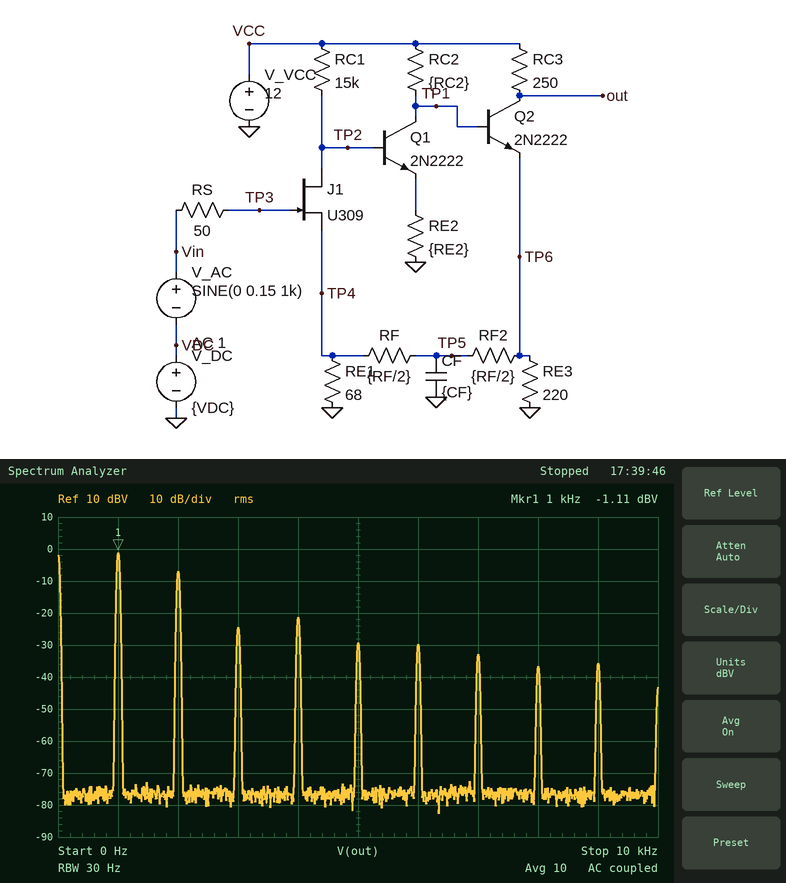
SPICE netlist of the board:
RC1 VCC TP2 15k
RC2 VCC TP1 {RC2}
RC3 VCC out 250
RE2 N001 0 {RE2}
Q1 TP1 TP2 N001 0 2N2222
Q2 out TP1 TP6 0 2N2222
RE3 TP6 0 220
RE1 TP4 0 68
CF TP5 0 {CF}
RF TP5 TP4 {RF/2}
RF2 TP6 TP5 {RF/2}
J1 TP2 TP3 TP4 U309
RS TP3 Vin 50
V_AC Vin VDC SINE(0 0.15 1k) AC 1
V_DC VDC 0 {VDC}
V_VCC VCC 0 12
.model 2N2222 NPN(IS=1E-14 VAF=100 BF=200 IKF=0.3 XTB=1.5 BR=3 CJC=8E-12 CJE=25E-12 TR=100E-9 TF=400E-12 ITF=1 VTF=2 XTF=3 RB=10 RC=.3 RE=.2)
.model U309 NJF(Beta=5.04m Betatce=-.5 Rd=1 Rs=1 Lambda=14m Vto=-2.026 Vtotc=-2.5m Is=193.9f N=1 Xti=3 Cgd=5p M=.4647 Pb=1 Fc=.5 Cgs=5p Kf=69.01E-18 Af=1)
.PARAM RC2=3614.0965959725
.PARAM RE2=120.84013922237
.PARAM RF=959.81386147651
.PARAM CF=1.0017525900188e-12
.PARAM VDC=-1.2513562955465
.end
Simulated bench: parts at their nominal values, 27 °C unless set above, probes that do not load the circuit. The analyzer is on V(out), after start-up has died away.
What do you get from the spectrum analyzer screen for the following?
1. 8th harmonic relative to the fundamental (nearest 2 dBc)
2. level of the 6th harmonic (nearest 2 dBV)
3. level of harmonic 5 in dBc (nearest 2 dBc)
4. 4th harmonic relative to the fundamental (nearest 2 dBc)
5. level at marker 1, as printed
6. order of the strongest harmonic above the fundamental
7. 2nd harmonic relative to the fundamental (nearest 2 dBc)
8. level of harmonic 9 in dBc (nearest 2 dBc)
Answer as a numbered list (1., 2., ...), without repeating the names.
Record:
1. -36 dBc
2. -30 dBV
3. -28 dBc
4. -20 dBc
5. -1.11 dBV
6. 2
7. -6 dBc
8. -34 dBc
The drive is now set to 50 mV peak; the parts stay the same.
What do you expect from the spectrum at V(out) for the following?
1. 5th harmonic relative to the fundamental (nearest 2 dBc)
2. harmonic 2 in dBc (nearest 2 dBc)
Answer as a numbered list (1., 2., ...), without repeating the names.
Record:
1. -18 dBc
2. -2 dBc
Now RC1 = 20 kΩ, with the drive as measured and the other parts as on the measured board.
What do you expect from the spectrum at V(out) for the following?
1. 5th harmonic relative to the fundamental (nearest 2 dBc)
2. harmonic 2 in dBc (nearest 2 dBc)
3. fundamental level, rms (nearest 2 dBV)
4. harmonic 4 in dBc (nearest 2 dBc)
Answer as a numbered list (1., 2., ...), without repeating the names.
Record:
1. -26 dBc
2. -2 dBc
3. -10 dBV
4. -16 dBc
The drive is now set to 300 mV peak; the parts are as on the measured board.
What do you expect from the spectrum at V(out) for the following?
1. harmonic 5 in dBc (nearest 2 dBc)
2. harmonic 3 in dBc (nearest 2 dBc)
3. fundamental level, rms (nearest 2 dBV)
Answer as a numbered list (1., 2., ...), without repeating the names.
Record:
1. -34 dBc
2. -30 dBc
3. 6 dBV
